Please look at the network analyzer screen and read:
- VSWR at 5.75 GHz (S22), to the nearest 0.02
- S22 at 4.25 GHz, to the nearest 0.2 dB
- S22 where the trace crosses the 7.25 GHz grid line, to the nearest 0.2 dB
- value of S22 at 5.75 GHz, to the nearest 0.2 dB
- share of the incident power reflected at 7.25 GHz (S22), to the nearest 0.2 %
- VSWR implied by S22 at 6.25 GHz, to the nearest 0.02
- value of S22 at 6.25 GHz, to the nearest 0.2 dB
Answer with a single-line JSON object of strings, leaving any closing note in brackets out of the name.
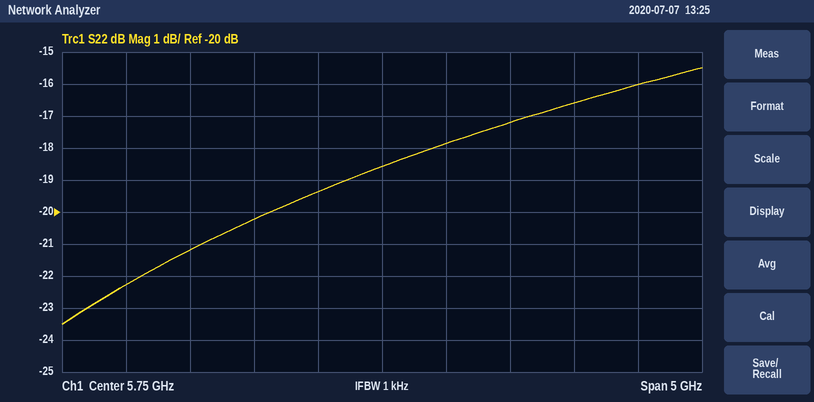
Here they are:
{"VSWR at 5.75 GHz (S22), to the nearest 0.02": "1.26", "S22 at 4.25 GHz, to the nearest 0.2 dB": "-21.2 dB", "S22 where the trace crosses the 7.25 GHz grid line, to the nearest 0.2 dB": "-16.6 dB", "value of S22 at 5.75 GHz, to the nearest 0.2 dB": "-18.6 dB", "share of the incident power reflected at 7.25 GHz (S22), to the nearest 0.2 %": "2.2 %", "VSWR implied by S22 at 6.25 GHz, to the nearest 0.02": "1.30", "value of S22 at 6.25 GHz, to the nearest 0.2 dB": "-17.8 dB"}
